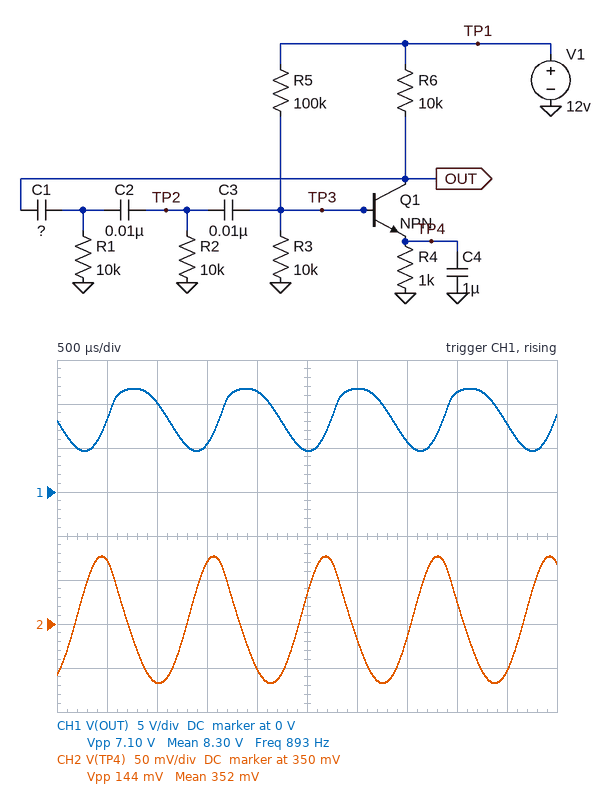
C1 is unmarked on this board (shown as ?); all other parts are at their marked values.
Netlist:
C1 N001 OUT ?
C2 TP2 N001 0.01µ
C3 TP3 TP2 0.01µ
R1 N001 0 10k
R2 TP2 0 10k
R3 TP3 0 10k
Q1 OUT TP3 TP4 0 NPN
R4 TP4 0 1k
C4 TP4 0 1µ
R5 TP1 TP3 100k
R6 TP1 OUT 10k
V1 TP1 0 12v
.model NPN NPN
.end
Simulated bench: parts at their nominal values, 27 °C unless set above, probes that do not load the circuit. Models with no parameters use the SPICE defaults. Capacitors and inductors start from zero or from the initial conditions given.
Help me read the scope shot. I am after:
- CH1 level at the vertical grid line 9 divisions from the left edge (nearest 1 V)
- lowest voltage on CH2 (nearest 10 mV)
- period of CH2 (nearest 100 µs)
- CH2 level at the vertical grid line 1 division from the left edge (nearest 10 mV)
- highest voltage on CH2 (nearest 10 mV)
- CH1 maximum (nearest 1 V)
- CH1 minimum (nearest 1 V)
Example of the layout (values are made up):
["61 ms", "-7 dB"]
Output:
["8 V", "280 mV", "1.1 ms", "420 mV", "430 mV", "12 V", "5 V"]
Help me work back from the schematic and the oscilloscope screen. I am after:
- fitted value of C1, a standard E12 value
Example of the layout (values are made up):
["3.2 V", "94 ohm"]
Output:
["5.6 nF"]
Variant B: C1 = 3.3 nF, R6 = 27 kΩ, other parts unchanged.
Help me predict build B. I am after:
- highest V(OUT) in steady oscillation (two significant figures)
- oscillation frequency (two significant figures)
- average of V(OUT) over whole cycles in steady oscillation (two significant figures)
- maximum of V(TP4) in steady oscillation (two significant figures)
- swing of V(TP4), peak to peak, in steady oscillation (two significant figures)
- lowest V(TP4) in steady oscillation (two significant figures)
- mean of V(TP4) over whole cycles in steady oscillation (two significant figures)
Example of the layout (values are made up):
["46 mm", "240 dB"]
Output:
["8.0 V", "870 Hz", "4.1 V", "330 mV", "63 mV", "270 mV", "300 mV"]
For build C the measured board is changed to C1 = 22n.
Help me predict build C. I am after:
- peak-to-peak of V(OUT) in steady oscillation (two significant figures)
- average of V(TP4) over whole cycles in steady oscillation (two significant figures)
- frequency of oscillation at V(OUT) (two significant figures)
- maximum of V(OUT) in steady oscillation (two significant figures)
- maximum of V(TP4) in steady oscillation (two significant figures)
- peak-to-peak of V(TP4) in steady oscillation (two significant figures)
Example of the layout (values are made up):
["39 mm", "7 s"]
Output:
["5.3 V", "340 mV", "640 Hz", "11 V", "440 mV", "190 mV"]
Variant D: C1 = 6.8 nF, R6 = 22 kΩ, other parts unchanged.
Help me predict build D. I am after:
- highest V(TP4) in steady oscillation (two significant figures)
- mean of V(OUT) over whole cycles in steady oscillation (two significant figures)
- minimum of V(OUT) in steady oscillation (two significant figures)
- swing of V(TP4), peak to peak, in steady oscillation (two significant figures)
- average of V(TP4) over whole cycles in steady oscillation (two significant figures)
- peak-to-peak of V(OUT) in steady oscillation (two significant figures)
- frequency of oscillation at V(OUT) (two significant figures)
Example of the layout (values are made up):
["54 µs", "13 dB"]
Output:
["370 mV", "5.5 V", "360 mV", "130 mV", "300 mV", "10 V", "760 Hz"]
